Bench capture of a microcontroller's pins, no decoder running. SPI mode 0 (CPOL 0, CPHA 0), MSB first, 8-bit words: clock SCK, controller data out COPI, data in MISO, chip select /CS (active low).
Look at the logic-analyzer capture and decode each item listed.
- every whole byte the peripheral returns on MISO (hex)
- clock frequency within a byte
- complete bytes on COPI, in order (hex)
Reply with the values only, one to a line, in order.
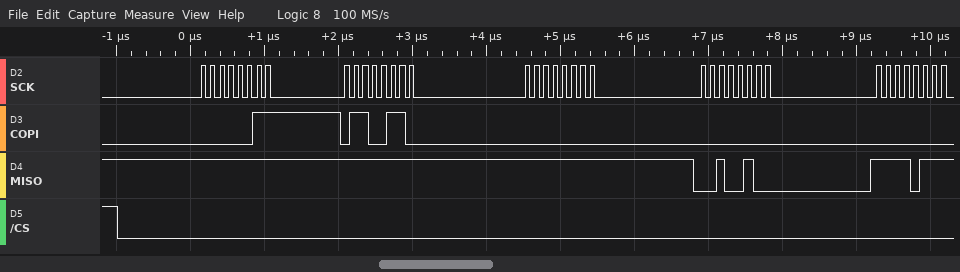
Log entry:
0xFF 0xFF 0xFF 0x24 0xF7
8 MHz
0x03 0x66 0x00 0x00 0x00
